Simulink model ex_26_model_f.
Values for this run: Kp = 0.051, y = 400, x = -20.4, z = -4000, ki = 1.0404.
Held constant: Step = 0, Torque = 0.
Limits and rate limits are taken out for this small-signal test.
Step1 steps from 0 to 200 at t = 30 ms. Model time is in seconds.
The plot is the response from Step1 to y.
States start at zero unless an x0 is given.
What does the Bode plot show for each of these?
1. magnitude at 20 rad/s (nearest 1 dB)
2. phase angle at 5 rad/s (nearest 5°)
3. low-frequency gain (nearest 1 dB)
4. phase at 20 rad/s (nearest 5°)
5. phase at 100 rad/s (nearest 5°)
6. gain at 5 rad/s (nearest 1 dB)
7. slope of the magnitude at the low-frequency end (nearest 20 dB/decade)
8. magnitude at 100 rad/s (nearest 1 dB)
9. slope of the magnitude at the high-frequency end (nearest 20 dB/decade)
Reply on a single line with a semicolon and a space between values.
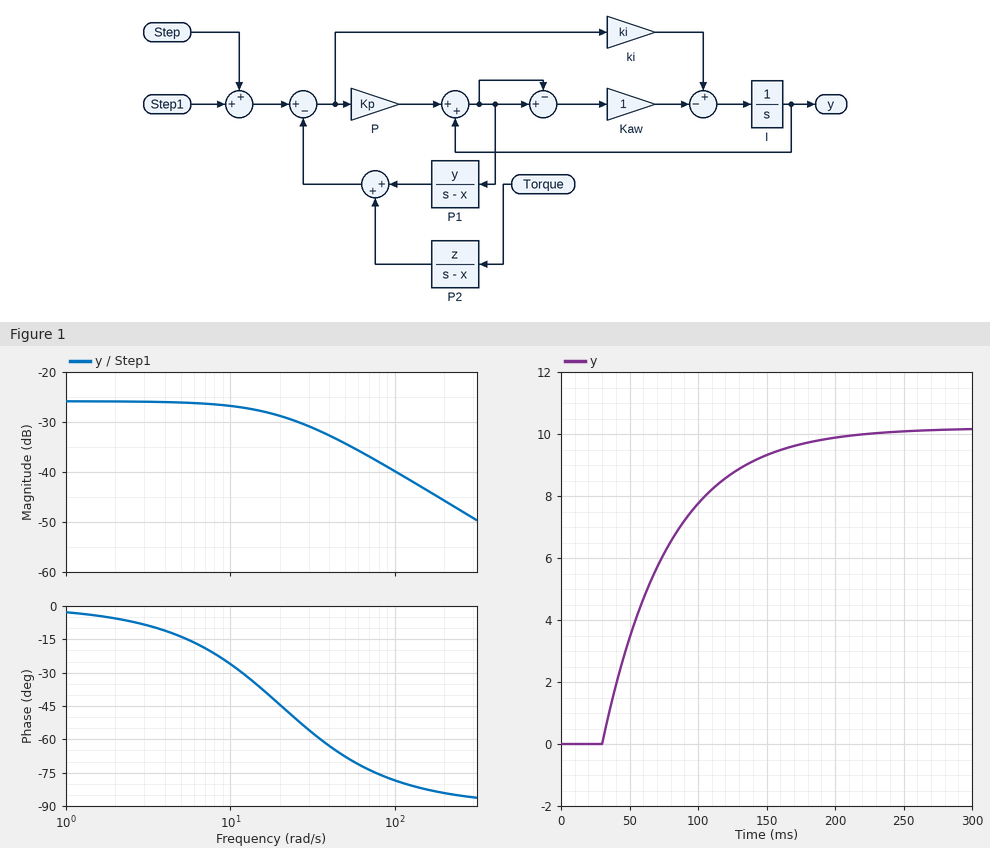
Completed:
-29 dB; -15°; -26 dB; -45°; -80°; -26 dB; 0 dB/decade; -40 dB; -20 dB/decade
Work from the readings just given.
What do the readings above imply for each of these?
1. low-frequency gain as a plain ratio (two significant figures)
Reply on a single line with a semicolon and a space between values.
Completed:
0.050
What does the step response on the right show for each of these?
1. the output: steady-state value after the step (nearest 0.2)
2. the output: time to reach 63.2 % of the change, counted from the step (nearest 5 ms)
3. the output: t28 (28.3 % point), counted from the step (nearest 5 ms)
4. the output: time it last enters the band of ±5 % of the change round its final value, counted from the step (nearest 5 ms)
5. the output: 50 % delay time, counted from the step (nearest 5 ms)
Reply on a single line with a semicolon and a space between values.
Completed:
10.2; 50 ms; 15 ms; 145 ms; 35 ms
